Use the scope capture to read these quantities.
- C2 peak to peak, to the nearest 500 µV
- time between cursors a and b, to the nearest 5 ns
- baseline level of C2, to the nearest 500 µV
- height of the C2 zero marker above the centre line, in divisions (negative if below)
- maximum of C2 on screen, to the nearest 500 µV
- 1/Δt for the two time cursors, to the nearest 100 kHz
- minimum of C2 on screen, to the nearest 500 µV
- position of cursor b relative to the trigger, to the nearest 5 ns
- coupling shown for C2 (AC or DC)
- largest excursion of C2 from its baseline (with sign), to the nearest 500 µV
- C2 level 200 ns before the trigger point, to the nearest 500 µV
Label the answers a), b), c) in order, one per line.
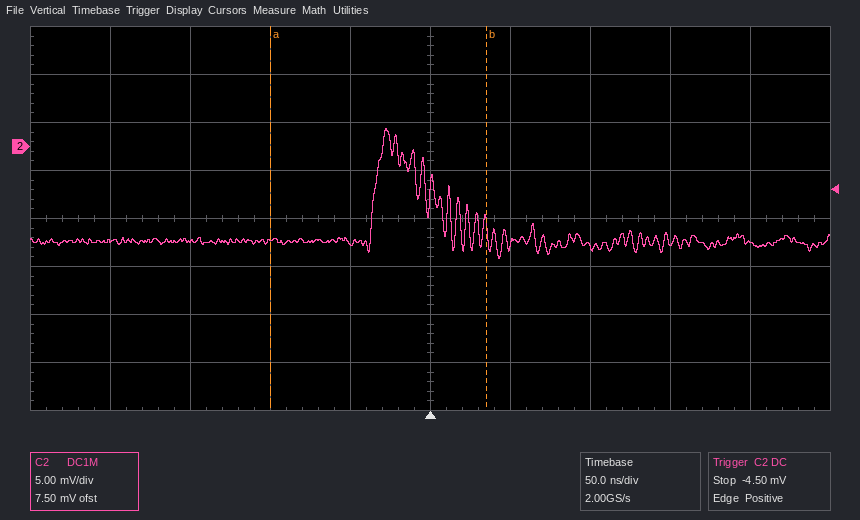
a) 13.5 mV
b) 135 ns
c) -10.0 mV
d) +1.5 div
e) 2.0 mV
f) 7.4 MHz
g) -11.5 mV
h) +35 ns
i) DC
j) +12.0 mV
k) -10.0 mV
